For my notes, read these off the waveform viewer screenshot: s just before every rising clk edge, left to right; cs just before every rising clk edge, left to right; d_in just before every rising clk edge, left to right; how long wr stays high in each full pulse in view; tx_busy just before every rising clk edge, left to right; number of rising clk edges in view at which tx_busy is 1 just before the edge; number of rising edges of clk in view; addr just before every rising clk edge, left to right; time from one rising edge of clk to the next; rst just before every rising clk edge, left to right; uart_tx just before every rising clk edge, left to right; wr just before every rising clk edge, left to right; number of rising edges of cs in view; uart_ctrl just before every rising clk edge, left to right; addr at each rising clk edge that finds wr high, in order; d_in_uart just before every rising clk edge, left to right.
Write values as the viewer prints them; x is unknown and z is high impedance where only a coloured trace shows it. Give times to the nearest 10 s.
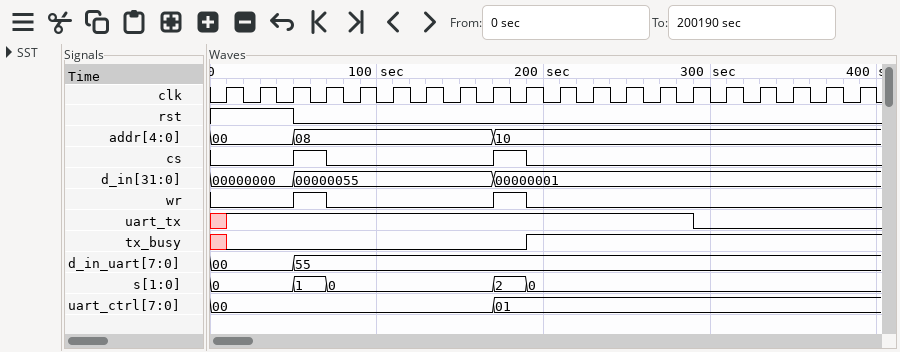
0, 0, 0, 1, 0, 0, 0, 0, 0, 2, 0, 0, 0, 0, 0, 0, 0, 0, 0, 0
0 0 0 1 0 0 0 0 0 1 0 0 0 0 0 0 0 0 0 0
00000000, 00000000, 00000000, 00000055, 00000055, 00000055, 00000055, 00000055, 00000055, 00000001, 00000001, 00000001, 00000001, 00000001, 00000001, 00000001, 00000001, 00000001, 00000001, 00000001
20 s, 20 s
x 0 0 0 0 0 0 0 0 0 1 1 1 1 1 1 1 1 1 1
10
20
00, 00, 00, 08, 08, 08, 08, 08, 08, 10, 10, 10, 10, 10, 10, 10, 10, 10, 10, 10
20 s
1 1 1 0 0 0 0 0 0 0 0 0 0 0 0 0 0 0 0 0
x 1 1 1 1 1 1 1 1 1 1 1 1 1 1 0 0 0 0 0
0 0 0 1 0 0 0 0 0 1 0 0 0 0 0 0 0 0 0 0
2
00, 00, 00, 00, 00, 00, 00, 00, 00, 01, 01, 01, 01, 01, 01, 01, 01, 01, 01, 01
08, 10
00, 00, 00, 55, 55, 55, 55, 55, 55, 55, 55, 55, 55, 55, 55, 55, 55, 55, 55, 55
